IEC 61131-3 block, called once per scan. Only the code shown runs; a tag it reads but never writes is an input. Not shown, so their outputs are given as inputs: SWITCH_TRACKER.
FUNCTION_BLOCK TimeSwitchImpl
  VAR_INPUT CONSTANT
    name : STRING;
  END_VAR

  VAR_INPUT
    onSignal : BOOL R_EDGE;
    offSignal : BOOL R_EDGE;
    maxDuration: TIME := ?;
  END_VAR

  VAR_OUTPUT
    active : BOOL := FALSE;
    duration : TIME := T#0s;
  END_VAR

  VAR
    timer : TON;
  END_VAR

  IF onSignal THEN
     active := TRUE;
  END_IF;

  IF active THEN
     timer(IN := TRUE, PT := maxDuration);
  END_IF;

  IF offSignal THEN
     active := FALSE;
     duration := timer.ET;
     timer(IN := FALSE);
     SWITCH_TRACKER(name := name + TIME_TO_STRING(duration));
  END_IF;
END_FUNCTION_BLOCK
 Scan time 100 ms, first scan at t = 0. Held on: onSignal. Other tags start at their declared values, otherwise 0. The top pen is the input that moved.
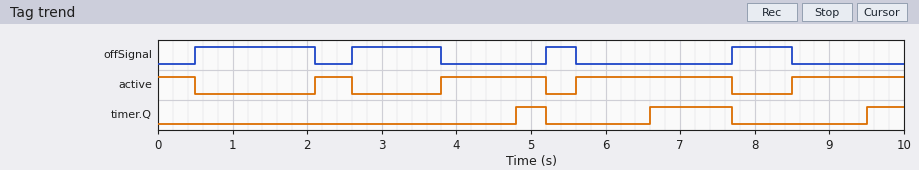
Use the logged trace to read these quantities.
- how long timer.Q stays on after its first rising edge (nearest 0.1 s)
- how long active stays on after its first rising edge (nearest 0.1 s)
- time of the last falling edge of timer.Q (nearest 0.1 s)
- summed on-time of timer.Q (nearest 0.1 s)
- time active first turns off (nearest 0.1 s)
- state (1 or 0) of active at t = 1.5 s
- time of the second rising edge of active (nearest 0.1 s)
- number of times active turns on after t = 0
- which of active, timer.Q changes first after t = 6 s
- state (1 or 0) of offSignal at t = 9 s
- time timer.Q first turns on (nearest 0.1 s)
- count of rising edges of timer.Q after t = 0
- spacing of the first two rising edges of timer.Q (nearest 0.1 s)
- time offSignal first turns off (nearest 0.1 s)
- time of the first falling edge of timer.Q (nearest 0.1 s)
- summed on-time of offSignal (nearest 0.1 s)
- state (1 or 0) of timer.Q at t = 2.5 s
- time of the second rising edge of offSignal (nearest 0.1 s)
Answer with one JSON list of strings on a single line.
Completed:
["0.4 s", "0.5 s", "7.7 s", "2.0 s", "0.5 s", "0", "3.8 s", "4", "timer.Q", "0", "4.8 s", "3", "1.8 s", "2.1 s", "5.2 s", "4.0 s", "0", "2.6 s"]
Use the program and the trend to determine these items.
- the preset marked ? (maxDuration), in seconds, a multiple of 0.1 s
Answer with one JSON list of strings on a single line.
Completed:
["1.0 s"]
